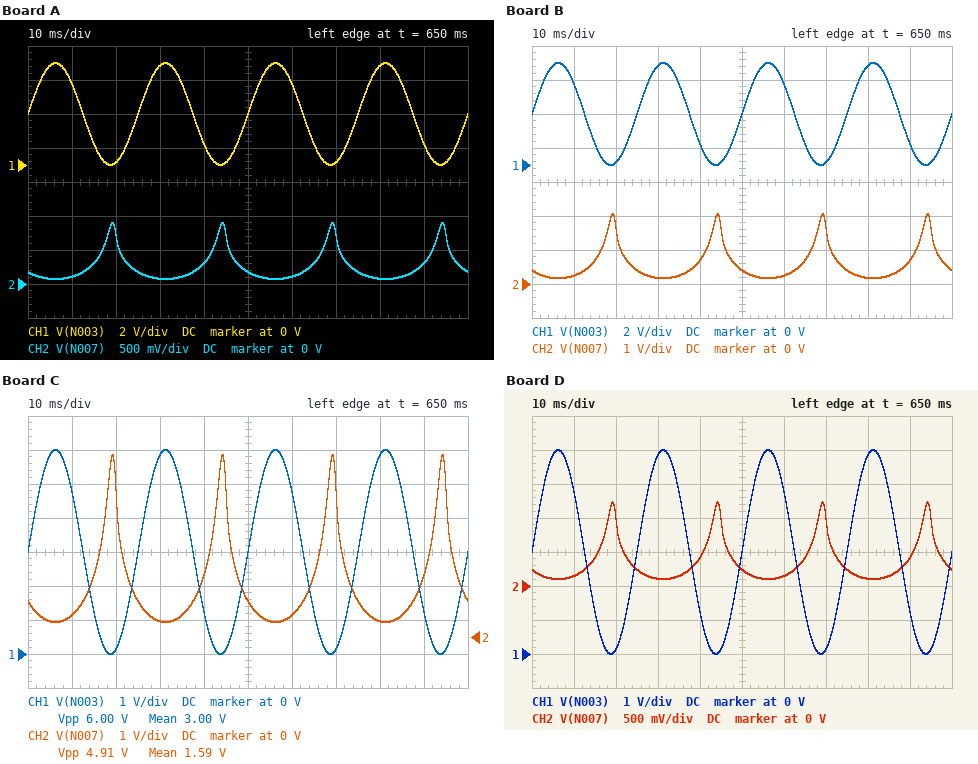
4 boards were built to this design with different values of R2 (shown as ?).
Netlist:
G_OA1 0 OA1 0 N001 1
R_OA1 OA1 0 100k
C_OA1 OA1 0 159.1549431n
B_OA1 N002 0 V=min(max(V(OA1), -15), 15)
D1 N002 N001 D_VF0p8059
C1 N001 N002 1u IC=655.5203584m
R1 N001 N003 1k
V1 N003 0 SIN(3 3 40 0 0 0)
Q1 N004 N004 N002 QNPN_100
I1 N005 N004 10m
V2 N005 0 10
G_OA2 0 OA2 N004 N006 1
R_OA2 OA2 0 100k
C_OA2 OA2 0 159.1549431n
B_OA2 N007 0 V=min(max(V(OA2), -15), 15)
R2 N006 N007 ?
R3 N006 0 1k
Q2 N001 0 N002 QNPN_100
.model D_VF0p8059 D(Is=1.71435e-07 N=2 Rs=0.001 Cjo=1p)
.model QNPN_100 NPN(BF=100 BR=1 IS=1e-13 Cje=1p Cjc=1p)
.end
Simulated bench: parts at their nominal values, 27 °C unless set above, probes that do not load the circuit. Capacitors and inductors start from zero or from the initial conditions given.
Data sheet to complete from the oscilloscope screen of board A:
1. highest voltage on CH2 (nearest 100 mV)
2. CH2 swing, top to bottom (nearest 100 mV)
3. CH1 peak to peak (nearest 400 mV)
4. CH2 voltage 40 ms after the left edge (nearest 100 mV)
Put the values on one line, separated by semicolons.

900 mV; 800 mV; 6.0 V; 300 mV
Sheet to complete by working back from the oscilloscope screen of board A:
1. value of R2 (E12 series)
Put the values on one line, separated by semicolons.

4.7 kΩ
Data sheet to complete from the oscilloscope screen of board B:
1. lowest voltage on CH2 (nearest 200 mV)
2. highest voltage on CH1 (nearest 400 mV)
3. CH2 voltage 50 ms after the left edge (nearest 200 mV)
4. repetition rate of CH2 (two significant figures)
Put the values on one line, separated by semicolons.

200 mV; 6.0 V; 400 mV; 40 Hz
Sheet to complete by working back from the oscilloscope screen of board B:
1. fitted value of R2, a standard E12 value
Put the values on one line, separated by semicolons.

12 kΩ
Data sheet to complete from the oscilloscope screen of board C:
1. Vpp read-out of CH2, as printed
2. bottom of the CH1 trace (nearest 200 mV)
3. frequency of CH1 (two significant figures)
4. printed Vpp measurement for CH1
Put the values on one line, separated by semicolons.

4.91 V; 0 V; 40 Hz; 6.00 V
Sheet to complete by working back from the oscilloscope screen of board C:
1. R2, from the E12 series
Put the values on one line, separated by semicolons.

33 kΩ
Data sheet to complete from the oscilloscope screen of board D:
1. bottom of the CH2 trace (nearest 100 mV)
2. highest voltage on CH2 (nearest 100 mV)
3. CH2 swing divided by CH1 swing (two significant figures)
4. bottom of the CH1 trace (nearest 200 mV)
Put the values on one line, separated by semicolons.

100 mV; 1.2 V; 0.19; 0 V
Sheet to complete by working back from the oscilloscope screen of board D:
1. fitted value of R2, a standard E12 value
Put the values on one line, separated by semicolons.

6.8 kΩ
